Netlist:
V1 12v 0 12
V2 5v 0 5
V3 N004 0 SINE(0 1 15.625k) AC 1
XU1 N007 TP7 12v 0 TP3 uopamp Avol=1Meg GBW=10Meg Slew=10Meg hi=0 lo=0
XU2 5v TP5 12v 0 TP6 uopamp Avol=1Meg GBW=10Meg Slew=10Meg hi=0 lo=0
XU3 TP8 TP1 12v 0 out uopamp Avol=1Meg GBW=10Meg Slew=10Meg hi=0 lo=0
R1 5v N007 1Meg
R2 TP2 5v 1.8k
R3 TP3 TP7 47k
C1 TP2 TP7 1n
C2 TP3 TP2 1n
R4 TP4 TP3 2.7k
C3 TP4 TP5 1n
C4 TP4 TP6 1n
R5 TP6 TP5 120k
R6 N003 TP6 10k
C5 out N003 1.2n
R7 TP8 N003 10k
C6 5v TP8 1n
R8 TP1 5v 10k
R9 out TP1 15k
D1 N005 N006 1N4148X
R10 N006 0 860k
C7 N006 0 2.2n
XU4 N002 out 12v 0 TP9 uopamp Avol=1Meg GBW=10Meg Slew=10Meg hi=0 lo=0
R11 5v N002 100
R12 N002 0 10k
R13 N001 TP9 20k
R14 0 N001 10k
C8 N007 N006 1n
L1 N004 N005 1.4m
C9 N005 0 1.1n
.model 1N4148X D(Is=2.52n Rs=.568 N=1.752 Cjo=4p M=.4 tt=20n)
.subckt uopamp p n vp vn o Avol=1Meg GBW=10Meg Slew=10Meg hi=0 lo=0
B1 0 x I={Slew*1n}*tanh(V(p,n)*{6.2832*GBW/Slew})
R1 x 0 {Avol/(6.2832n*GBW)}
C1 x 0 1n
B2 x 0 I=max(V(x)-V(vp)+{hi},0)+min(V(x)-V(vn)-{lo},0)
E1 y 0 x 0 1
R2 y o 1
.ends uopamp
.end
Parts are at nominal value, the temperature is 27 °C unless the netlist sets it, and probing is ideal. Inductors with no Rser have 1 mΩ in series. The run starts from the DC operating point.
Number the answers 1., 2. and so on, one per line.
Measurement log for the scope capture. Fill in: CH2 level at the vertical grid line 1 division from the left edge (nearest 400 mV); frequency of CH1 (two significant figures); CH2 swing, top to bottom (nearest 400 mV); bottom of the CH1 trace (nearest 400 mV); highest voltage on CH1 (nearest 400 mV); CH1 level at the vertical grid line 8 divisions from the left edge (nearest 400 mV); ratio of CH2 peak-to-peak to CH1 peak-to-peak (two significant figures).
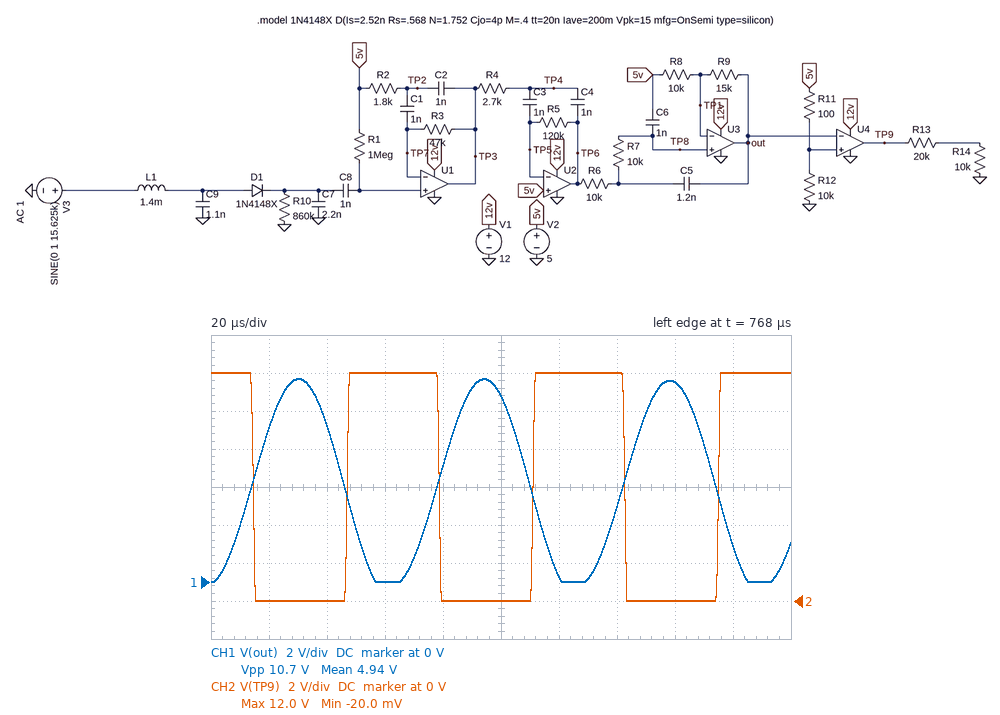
1. 0 V
2. 16 kHz
3. 12.0 V
4. 0 V
5. 10.8 V
6. 10.4 V
7. 1.1
